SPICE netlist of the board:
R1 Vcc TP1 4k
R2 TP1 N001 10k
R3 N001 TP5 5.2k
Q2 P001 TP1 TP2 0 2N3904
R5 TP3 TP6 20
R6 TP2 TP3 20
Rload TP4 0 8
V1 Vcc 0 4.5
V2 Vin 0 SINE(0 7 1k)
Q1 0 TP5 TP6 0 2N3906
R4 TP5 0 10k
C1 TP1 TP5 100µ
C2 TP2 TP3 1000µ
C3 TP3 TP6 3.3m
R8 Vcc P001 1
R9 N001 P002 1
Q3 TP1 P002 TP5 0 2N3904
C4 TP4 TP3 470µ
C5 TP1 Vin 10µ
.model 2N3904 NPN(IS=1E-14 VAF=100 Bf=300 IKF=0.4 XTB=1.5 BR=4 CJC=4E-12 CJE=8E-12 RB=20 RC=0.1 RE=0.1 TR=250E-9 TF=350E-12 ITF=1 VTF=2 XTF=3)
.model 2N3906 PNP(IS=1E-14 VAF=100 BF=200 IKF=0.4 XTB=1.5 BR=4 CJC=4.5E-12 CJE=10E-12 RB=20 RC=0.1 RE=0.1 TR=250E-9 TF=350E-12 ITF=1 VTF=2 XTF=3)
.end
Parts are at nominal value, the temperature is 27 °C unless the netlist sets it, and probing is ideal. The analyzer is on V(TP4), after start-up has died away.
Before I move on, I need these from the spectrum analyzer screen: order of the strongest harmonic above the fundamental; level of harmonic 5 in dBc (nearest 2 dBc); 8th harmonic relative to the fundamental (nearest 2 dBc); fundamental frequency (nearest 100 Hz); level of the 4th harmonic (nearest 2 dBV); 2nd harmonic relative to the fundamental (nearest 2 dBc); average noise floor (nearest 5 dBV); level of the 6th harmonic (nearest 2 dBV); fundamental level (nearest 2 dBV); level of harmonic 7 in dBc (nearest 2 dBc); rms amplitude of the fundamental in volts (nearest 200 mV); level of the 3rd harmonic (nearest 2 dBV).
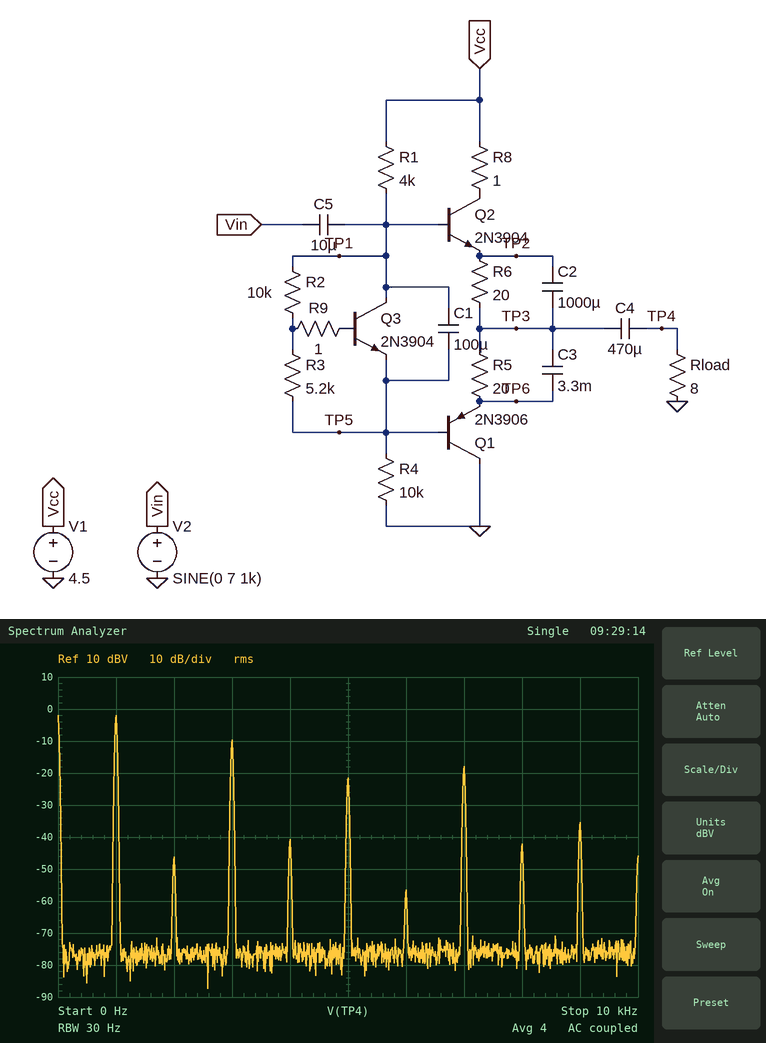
3
-20 dBc
-40 dBc
1.0 kHz
-40 dBV
-44 dBc
-75 dBV
-56 dBV
-2 dBV
-16 dBc
800 mV
-10 dBV
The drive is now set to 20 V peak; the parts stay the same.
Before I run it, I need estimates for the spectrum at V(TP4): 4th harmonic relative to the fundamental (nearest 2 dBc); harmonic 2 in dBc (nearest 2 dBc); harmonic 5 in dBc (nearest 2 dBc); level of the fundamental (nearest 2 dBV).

-52 dBc
-52 dBc
-20 dBc
-2 dBV
